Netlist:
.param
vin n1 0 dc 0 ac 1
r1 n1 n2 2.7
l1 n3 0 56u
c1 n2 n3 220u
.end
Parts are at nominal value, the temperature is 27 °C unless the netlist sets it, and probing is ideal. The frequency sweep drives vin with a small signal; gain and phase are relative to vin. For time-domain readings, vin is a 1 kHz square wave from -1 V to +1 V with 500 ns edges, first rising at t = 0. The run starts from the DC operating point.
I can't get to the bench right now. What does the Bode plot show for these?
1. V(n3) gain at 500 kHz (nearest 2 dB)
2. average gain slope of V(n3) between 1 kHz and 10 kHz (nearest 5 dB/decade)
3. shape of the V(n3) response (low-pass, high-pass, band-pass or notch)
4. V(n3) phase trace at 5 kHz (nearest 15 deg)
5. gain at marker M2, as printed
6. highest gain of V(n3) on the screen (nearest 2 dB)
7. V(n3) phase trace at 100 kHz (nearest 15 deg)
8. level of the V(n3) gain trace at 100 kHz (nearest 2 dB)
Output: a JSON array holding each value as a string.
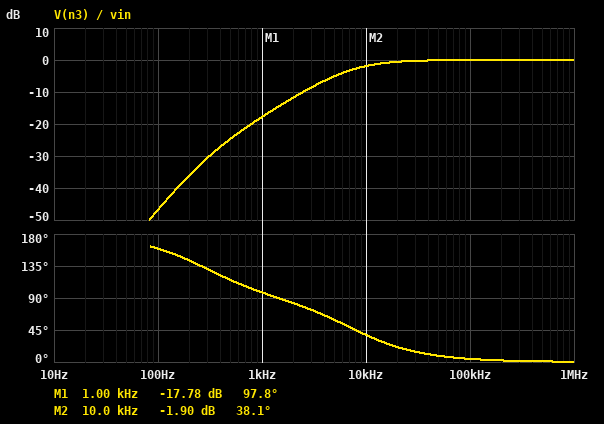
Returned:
["0 dB", "15 dB/decade", "high-pass", "60 deg", "-1.90 dB", "0 dB", "0 deg", "0 dB"]
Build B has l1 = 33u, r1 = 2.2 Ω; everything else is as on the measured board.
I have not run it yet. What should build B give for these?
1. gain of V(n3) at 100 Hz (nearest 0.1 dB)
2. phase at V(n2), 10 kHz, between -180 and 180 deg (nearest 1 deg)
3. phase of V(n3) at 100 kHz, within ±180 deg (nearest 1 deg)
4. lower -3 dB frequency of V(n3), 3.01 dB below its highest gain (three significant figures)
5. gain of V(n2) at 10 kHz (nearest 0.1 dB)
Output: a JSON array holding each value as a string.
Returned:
["-51.2 dB", "48 deg", "6 deg", "10.3 kHz", "-3.4 dB"]
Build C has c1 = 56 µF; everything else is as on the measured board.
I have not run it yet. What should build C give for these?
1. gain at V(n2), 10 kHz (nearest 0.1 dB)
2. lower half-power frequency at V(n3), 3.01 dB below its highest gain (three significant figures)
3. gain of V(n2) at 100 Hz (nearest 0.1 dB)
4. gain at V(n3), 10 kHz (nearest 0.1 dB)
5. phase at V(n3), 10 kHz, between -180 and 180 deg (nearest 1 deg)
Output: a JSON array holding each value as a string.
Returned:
["-2.3 dB", "6.65 kHz", "0 dB", "-1.6 dB", "40 deg"]
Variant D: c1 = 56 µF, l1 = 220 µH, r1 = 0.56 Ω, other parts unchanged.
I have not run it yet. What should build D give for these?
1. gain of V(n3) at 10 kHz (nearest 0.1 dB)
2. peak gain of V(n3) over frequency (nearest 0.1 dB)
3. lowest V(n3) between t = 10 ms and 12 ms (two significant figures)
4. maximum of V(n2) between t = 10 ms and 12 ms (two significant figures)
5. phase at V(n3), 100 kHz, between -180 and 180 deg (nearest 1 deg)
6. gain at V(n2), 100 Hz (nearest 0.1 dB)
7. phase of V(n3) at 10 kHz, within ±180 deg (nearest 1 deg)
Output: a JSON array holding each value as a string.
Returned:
["0.2 dB", "11.1 dB", "-1.6 V", "1.3 V", "0 deg", "0 dB", "2 deg"]
